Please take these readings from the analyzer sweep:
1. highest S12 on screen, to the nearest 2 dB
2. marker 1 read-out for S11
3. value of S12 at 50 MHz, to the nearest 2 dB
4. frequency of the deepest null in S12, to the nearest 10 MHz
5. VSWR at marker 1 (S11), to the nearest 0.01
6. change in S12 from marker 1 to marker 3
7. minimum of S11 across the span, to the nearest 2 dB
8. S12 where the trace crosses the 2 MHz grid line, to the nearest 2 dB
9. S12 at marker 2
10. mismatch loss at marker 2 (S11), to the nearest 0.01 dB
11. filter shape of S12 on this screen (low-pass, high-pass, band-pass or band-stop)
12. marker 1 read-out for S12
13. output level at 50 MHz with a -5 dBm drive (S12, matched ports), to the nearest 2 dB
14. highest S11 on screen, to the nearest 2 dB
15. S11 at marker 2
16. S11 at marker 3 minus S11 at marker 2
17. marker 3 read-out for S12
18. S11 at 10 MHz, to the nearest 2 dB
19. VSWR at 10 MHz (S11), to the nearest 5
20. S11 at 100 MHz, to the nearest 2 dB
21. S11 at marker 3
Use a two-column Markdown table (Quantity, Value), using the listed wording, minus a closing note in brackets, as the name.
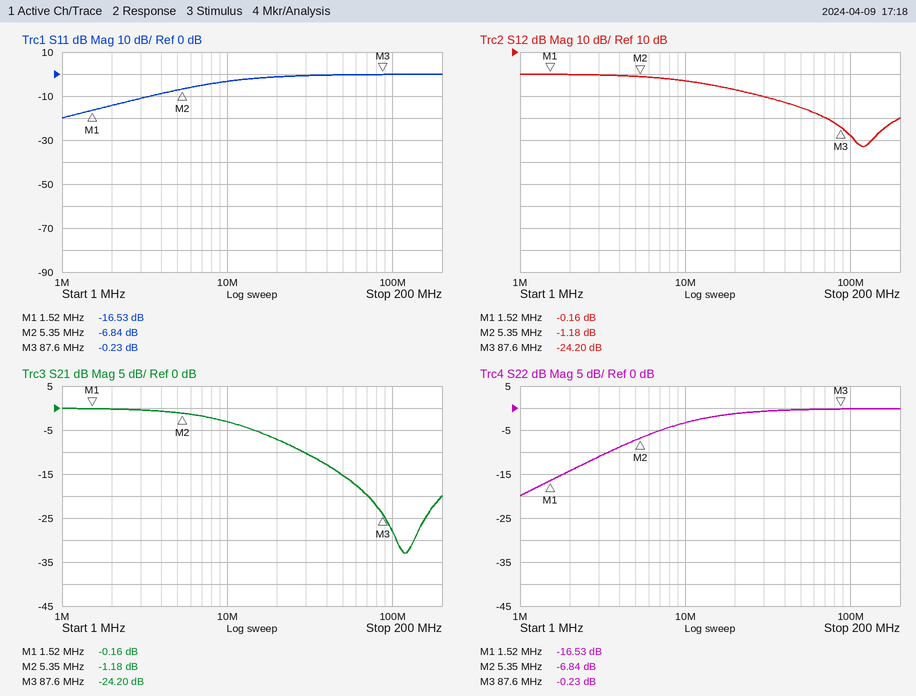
| Quantity | Value |
|---|---|
| highest S12 on screen, to the nearest 2 dB | 0 dB |
| marker 1 read-out for S11 | -16.53 dB |
| value of S12 at 50 MHz, to the nearest 2 dB | -16 dB |
| frequency of the deepest null in S12, to the nearest 10 MHz | 120 MHz |
| VSWR at marker 1 (S11), to the nearest 0.01 | 1.35 |
| change in S12 from marker 1 to marker 3 | -24.04 dB |
| minimum of S11 across the span, to the nearest 2 dB | -20 dB |
| S12 where the trace crosses the 2 MHz grid line, to the nearest 2 dB | 0 dB |
| S12 at marker 2 | -1.18 dB |
| mismatch loss at marker 2 (S11), to the nearest 0.01 dB | 1.01 dB |
| filter shape of S12 on this screen | low-pass |
| marker 1 read-out for S12 | -0.16 dB |
| output level at 50 MHz with a -5 dBm drive (S12, matched ports), to the nearest 2 dB | -20 dBm |
| highest S11 on screen, to the nearest 2 dB | 0 dB |
| S11 at marker 2 | -6.84 dB |
| S11 at marker 3 minus S11 at marker 2 | 6.61 dB |
| marker 3 read-out for S12 | -24.20 dB |
| S11 at 10 MHz, to the nearest 2 dB | -4 dB |
| VSWR at 10 MHz (S11), to the nearest 5 | 5 |
| S11 at 100 MHz, to the nearest 2 dB | 0 dB |
| S11 at marker 3 | -0.23 dB |
